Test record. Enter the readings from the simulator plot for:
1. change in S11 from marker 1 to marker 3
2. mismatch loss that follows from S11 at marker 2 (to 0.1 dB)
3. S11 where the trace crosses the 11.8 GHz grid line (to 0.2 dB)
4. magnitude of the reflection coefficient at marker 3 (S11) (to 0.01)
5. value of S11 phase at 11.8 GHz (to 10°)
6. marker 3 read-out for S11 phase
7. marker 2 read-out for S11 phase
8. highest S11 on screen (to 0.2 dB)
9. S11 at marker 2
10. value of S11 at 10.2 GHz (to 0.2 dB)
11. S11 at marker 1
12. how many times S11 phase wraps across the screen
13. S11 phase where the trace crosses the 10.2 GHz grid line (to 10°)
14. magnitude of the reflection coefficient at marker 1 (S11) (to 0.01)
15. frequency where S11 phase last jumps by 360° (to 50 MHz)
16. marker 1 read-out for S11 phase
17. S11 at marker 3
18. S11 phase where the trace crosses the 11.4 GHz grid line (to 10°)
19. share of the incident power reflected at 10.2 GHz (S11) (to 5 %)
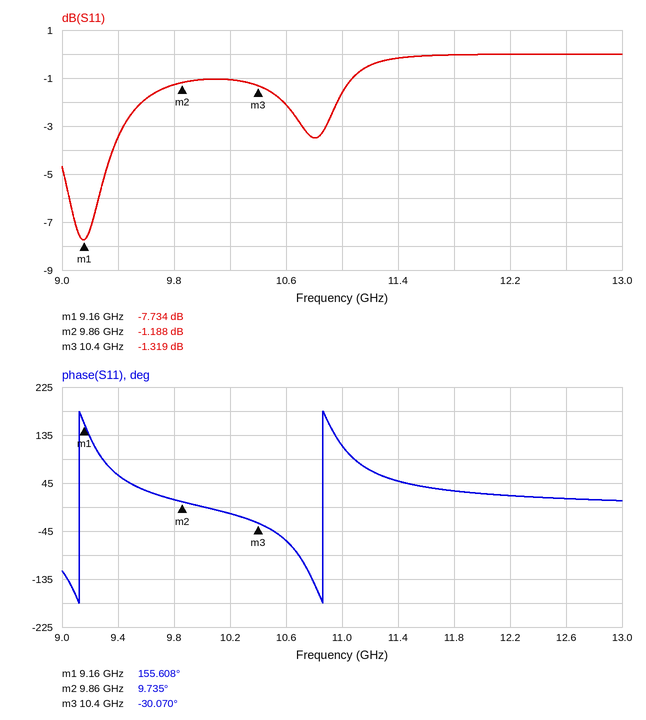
6.415 dB
6.2 dB
0.0 dB
0.86
30°
-30.070°
9.735°
0.0 dB
-1.188 dB
-1.0 dB
-7.734 dB
2
-10°
0.41
10.85 GHz
155.608°
-1.319 dB
50°
80 %
